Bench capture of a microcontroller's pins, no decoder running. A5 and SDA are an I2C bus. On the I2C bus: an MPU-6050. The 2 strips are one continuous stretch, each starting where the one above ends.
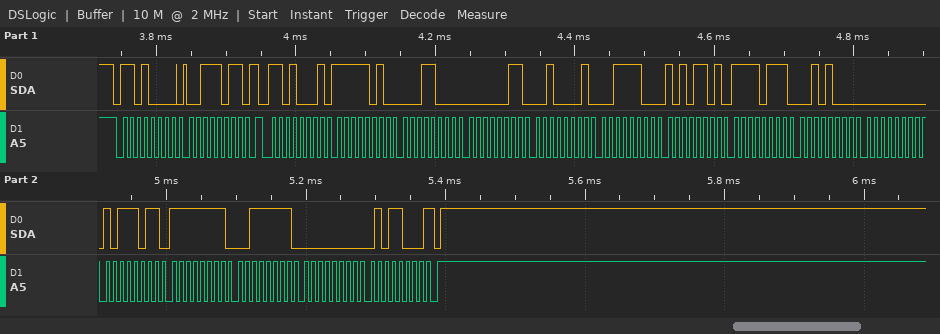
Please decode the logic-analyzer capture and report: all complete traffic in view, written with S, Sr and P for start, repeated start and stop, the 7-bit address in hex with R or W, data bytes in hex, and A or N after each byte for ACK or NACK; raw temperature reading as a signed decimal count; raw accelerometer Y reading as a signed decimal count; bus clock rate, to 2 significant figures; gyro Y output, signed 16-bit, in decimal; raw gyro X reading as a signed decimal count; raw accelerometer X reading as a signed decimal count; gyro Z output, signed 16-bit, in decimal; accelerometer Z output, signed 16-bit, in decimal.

S 68W A 3B A Sr 68R A FA A 18 A 03 A 21 A 3C A AD A F7 A 28 A 00 A BB A FF A 3F A 00 A 58 N P
-2264
801
100 kHz
-193
187
-1512
88
15533
